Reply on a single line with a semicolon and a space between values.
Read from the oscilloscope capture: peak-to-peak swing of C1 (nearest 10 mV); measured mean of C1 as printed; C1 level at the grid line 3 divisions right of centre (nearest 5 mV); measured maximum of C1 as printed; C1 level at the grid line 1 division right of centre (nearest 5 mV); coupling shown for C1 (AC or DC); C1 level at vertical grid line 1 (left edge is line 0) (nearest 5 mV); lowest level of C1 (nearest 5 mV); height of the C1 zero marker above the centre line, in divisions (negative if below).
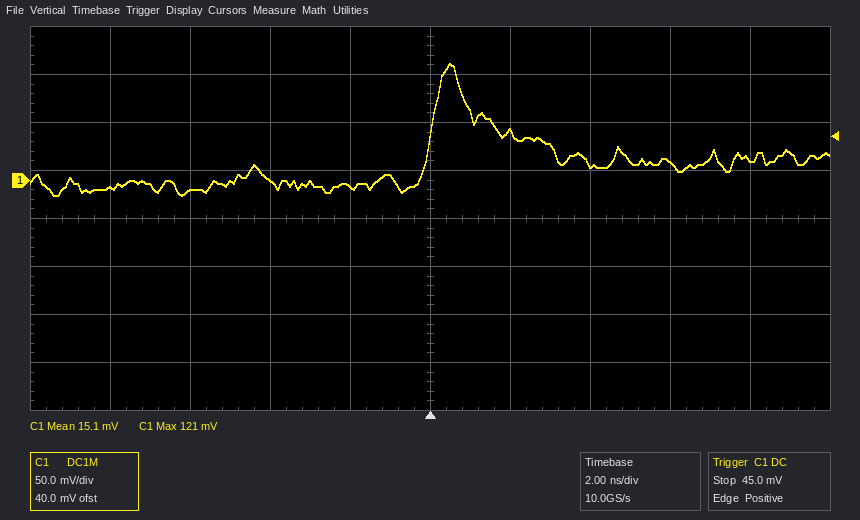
140 mV; 15.1 mV; 20 mV; 121 mV; 50 mV; DC; -10 mV; -15 mV; +0.8 div
